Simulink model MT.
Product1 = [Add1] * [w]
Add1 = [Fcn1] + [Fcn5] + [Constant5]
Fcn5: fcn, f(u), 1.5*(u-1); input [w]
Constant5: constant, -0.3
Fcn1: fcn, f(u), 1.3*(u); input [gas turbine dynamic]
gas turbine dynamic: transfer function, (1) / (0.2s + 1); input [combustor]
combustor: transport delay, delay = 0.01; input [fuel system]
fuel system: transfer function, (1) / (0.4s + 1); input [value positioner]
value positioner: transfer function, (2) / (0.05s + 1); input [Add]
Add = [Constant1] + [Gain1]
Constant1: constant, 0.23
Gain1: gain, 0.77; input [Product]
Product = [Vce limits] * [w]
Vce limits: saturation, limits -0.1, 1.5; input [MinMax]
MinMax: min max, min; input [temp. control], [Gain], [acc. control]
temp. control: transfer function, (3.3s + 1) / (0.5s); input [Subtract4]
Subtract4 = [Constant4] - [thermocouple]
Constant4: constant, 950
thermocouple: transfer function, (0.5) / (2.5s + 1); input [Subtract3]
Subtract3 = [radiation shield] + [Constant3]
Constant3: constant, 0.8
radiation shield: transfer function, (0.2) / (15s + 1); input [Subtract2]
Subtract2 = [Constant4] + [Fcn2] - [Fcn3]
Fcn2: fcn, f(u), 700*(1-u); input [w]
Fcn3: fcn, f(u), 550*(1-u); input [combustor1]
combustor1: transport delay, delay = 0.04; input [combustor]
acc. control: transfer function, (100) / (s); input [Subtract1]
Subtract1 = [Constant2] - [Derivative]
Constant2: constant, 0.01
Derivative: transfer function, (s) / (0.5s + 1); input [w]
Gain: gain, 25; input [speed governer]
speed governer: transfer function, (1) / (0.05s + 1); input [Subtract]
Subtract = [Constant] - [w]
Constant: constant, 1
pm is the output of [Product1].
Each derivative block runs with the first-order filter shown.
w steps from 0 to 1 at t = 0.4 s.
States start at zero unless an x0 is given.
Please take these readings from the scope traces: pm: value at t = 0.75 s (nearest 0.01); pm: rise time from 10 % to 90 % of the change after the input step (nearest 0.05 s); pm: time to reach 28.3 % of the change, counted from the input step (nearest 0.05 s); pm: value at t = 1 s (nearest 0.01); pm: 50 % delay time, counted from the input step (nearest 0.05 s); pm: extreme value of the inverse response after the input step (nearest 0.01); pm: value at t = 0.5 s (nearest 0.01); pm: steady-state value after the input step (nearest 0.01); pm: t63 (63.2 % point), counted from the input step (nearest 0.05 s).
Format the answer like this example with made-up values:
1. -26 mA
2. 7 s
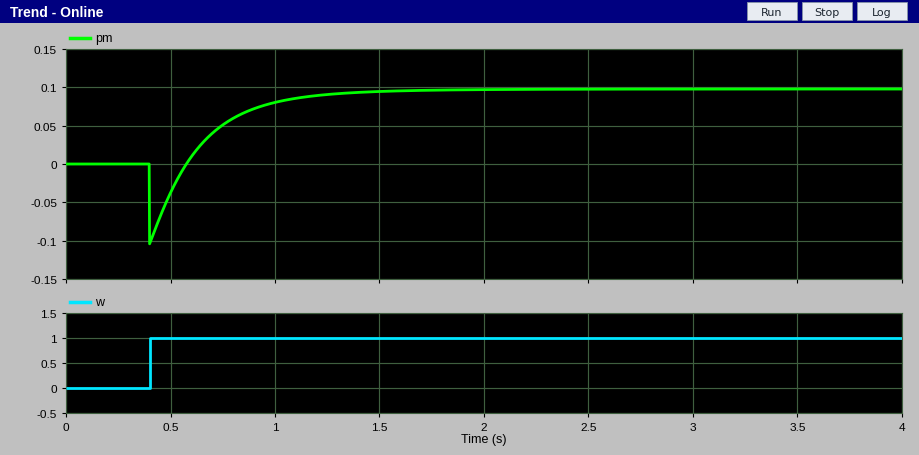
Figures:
1. 0.05
2. 0.55 s
3. 0.25 s
4. 0.08
5. 0.35 s
6. -0.10
7. -0.04
8. 0.10
9. 0.40 s
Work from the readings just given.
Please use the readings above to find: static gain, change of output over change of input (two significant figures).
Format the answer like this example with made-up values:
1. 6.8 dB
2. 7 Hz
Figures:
1. 0.10
